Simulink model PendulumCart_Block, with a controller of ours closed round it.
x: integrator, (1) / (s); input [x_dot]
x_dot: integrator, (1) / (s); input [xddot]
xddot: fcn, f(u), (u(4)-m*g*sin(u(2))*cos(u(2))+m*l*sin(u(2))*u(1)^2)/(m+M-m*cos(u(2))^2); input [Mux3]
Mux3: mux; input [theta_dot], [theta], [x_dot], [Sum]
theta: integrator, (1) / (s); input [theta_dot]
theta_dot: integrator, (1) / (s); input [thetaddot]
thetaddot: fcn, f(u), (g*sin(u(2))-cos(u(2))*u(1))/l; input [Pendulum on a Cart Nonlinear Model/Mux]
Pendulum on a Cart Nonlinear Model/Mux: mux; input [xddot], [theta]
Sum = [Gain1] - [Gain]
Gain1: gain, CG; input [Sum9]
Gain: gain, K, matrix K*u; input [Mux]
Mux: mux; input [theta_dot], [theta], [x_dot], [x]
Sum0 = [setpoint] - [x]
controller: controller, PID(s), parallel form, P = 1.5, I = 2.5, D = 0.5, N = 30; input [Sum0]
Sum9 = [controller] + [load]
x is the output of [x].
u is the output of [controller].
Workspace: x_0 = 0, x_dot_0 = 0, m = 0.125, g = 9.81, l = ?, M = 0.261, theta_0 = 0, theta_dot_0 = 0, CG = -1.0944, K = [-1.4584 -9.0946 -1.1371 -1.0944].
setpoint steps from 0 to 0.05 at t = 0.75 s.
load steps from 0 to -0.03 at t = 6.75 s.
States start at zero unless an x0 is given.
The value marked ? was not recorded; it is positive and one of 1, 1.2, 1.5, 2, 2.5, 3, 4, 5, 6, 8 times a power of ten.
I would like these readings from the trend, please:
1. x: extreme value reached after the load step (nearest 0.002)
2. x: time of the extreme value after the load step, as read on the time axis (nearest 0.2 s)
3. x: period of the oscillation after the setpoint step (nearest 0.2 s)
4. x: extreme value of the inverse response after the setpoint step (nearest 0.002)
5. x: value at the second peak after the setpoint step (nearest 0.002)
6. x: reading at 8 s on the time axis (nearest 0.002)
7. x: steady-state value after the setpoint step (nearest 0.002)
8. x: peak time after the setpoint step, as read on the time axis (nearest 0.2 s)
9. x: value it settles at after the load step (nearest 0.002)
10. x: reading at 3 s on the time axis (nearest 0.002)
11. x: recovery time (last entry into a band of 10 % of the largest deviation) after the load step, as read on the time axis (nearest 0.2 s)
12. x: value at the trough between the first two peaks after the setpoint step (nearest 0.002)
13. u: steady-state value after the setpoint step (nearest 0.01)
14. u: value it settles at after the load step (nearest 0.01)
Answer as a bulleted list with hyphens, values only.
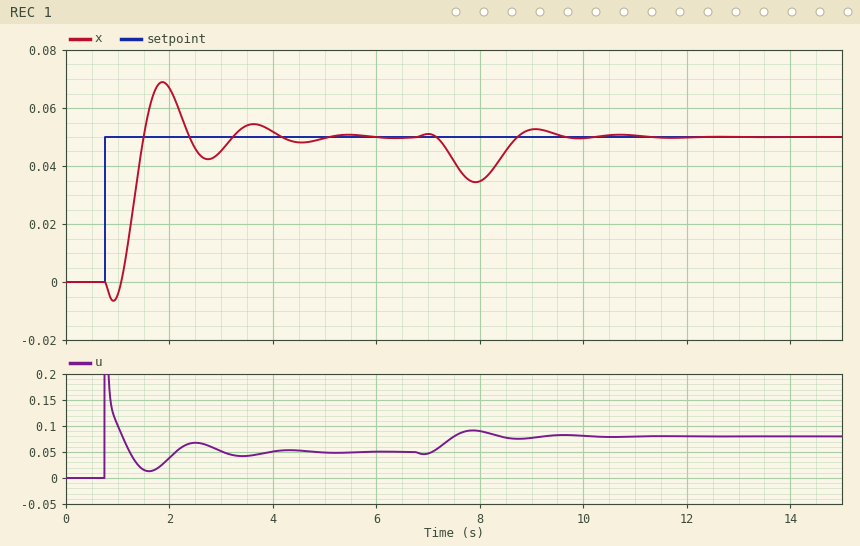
- 0.034
- 8.0 s
- 1.8 s
- -0.006
- 0.054
- 0.034
- 0.050
- 1.8 s
- 0.050
- 0.046
- 9.4 s
- 0.042
- 0.05
- 0.08
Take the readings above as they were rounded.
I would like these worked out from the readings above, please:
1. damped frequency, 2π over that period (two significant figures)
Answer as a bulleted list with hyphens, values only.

- 3.5 rad/s
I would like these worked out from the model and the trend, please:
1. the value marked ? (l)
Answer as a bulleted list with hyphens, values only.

- 0.3
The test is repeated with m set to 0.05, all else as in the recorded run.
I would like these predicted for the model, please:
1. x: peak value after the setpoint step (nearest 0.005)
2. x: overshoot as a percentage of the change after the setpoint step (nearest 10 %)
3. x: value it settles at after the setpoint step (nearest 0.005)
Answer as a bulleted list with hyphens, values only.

- 0.065
- 30 %
- 0.050
